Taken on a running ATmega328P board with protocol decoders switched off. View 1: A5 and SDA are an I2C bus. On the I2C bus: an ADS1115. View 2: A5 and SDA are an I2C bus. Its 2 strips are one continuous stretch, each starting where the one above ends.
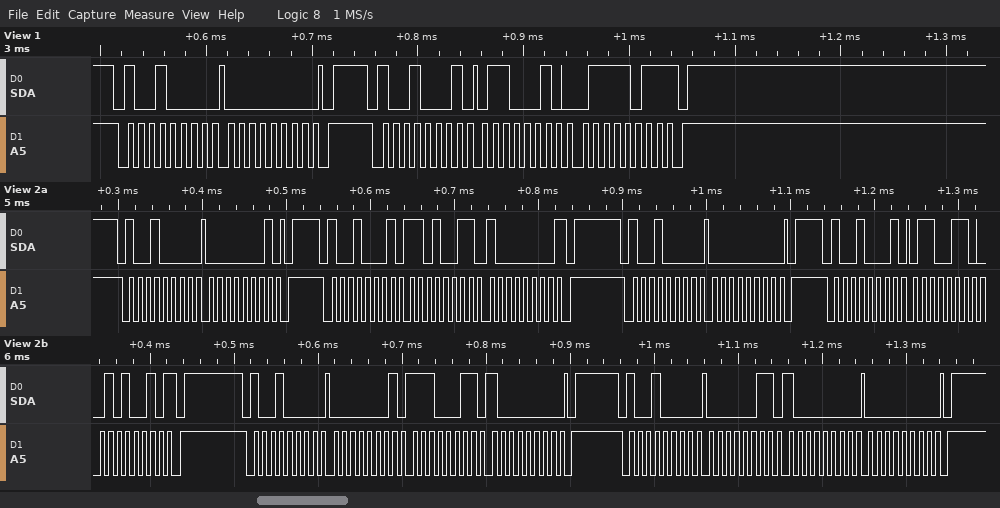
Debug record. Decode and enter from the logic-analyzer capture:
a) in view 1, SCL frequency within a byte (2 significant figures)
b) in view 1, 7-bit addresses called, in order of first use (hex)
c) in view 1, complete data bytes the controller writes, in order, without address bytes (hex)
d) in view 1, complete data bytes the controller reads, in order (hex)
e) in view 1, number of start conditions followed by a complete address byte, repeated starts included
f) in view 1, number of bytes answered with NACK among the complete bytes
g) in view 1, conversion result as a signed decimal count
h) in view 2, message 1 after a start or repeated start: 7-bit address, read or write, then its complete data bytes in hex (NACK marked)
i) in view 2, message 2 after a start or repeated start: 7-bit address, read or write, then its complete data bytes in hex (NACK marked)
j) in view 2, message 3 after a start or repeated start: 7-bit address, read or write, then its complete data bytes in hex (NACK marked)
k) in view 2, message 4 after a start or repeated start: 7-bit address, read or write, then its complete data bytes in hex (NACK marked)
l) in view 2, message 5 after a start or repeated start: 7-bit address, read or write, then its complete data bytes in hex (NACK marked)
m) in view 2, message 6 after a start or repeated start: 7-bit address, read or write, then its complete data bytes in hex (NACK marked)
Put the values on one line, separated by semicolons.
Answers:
100 kHz; 0x48; 00; 62 7B; 2; 1; 25211; 0x48 write: 01; 0x48 read: D3 80 NACK; 0x48 write: 00; 0x48 read: 66 52 NACK; 0x48 write: 01 E3 80; 0x48 write: 03 80 00
